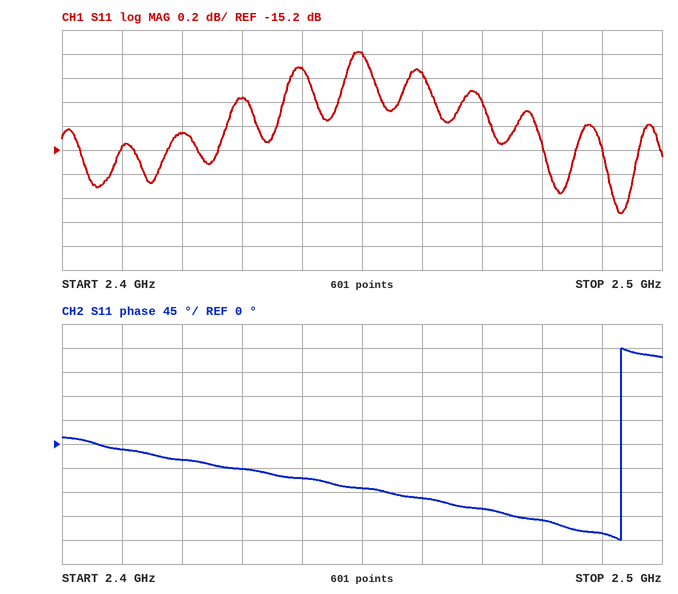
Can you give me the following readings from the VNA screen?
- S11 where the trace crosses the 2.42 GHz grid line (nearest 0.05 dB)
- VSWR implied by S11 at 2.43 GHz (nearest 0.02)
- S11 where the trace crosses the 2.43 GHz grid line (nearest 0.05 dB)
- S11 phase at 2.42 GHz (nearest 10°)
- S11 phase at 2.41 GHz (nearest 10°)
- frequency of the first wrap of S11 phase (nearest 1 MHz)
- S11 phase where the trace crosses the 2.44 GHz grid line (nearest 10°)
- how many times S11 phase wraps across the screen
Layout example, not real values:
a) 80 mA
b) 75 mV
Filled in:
a) -15.05 dB
b) 1.44
c) -14.75 dB
d) -30°
e) -10°
f) 2.493 GHz
g) -60°
h) 1
